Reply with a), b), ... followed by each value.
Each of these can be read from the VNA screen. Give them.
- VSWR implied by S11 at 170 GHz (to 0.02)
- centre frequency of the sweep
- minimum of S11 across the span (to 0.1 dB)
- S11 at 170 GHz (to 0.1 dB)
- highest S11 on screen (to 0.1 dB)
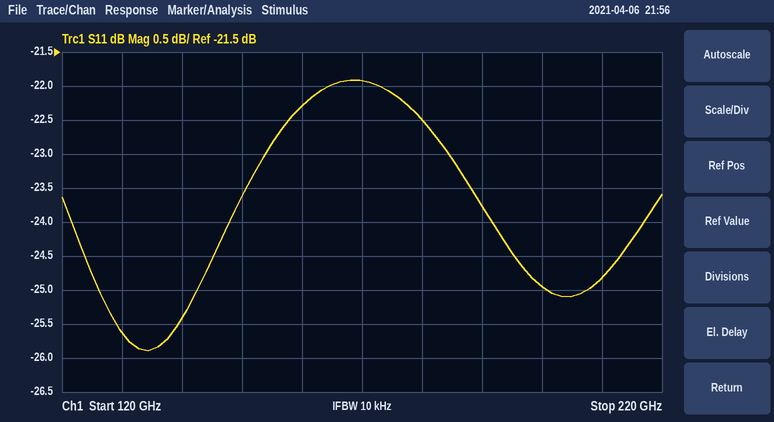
a) 1.18
b) 170 GHz
c) -25.9 dB
d) -21.9 dB
e) -21.9 dB
